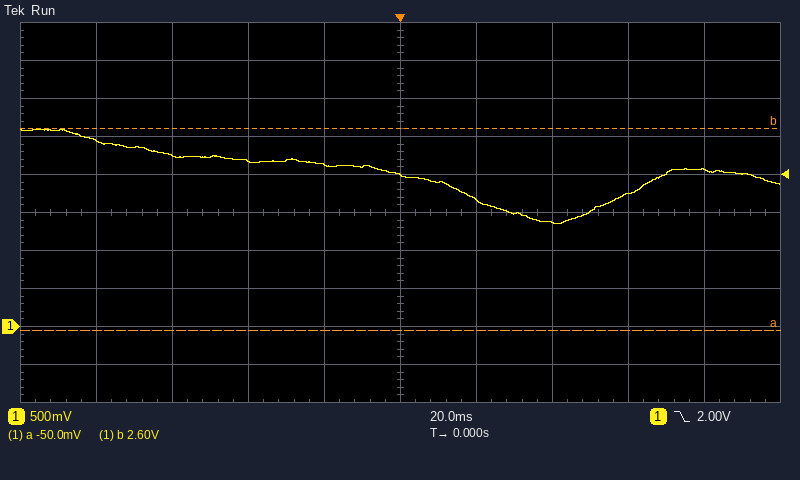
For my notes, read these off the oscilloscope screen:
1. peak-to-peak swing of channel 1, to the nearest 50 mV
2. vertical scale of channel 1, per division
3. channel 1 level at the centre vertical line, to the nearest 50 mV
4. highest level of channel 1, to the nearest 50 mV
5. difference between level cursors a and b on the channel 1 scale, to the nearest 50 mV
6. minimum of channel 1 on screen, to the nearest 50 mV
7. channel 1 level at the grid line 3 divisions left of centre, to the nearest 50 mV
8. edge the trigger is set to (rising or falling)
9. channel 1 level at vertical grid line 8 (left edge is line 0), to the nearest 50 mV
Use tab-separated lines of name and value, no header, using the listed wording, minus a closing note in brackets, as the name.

peak-to-peak swing of channel 1, to the nearest 50 mV	1.25 V
vertical scale of channel 1, per division	500 mV
channel 1 level at the centre vertical line, to the nearest 50 mV	2.00 V
highest level of channel 1, to the nearest 50 mV	2.60 V
difference between level cursors a and b on the channel 1 scale, to the nearest 50 mV	2.65 V
minimum of channel 1 on screen, to the nearest 50 mV	1.35 V
channel 1 level at the grid line 3 divisions left of centre, to the nearest 50 mV	2.25 V
edge the trigger is set to	falling
channel 1 level at vertical grid line 8 (left edge is line 0), to the nearest 50 mV	1.75 V
